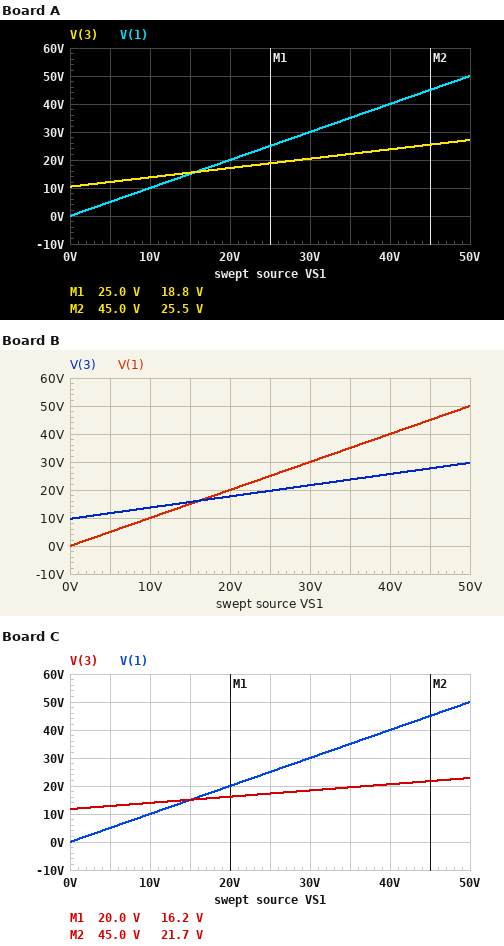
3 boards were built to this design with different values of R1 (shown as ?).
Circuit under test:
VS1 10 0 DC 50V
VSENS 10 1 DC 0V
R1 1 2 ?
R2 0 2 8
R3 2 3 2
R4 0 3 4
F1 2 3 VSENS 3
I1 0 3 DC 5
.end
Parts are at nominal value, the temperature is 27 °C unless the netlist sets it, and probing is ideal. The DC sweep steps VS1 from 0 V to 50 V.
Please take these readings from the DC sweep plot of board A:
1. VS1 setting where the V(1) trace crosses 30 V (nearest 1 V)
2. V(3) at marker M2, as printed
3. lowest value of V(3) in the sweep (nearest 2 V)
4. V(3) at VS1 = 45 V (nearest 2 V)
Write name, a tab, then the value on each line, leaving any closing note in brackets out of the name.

VS1 setting where the V(1) trace crosses 30 V	30 V
V(3) at marker M2, as printed	25.5 V
lowest value of V(3) in the sweep	10 V
V(3) at VS1 = 45 V	26 V
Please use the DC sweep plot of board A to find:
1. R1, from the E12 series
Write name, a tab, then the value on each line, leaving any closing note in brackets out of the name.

R1, from the E12 series	12 Ω
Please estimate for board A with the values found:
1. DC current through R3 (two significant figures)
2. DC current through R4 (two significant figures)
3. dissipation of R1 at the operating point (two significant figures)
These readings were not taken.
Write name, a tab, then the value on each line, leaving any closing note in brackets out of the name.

DC current through R3	7.9 A
DC current through R4	6.8 A
dissipation of R1 at the operating point	120 W
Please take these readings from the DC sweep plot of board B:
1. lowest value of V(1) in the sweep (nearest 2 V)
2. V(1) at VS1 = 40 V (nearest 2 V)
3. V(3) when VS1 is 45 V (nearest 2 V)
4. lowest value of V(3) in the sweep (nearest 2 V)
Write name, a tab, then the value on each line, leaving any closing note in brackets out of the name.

lowest value of V(1) in the sweep	0 V
V(1) at VS1 = 40 V	40 V
V(3) when VS1 is 45 V	28 V
lowest value of V(3) in the sweep	10 V
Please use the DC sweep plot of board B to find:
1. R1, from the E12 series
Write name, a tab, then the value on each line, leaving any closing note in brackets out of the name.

R1, from the E12 series	10 Ω
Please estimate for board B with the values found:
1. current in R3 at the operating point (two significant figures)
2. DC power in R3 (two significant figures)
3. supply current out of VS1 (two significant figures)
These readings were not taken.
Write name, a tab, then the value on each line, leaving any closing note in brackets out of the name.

current in R3 at the operating point	9.1 A
DC power in R3	170 W
supply current out of VS1	3.9 A
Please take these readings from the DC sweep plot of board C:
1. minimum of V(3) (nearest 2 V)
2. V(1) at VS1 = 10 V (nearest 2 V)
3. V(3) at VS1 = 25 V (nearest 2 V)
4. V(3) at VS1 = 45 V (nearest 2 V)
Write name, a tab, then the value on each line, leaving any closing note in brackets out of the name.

minimum of V(3)	12 V
V(1) at VS1 = 10 V	10 V
V(3) at VS1 = 25 V	18 V
V(3) at VS1 = 45 V	22 V
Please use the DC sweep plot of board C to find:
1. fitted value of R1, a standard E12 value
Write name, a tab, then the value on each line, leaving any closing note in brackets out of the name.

fitted value of R1, a standard E12 value	18 Ω
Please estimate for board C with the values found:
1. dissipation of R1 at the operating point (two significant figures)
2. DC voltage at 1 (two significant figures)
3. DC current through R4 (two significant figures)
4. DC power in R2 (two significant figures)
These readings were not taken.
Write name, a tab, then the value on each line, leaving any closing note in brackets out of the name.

dissipation of R1 at the operating point	83 W
DC voltage at 1	50 V
DC current through R4	5.7 A
DC power in R2	16 W
